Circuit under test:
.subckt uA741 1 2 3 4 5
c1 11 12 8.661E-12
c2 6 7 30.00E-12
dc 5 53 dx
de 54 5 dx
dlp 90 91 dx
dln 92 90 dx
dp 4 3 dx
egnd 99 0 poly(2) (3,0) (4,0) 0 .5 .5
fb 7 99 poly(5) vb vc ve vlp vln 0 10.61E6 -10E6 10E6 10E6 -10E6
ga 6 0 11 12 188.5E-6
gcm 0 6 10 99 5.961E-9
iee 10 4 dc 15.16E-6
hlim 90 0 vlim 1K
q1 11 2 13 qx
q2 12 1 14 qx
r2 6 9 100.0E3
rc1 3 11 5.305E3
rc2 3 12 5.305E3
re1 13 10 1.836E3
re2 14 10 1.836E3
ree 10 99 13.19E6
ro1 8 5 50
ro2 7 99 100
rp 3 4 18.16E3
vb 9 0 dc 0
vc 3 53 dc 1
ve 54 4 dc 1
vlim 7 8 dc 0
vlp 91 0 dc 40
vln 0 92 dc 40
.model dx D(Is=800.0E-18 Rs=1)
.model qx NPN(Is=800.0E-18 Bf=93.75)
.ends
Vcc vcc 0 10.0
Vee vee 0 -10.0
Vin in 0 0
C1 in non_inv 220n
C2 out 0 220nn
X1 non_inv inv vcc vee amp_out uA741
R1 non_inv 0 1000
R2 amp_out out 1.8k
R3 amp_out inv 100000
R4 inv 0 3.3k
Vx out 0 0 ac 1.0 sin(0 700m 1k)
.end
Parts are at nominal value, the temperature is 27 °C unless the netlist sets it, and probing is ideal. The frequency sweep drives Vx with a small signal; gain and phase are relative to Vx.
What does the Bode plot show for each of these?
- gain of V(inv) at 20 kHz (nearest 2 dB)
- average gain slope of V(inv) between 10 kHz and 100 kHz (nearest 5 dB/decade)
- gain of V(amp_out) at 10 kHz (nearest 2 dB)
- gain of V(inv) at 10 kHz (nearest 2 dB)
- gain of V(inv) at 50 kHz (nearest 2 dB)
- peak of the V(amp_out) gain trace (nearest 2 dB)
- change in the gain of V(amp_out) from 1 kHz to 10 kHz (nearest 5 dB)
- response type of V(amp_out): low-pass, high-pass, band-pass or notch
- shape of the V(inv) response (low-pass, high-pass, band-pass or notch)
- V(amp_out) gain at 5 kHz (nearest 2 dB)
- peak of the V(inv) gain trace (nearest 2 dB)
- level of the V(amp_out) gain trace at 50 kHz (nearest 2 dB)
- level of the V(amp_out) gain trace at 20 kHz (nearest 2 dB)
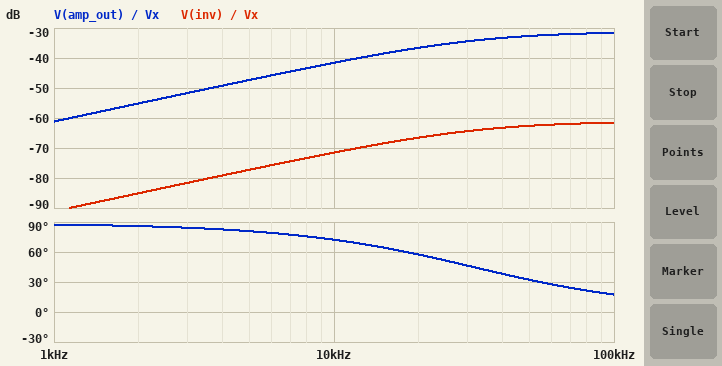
-66 dB
10 dB/decade
-42 dB
-72 dB
-62 dB
-32 dB
20 dB
high-pass
high-pass
-48 dB
-62 dB
-32 dB
-36 dB
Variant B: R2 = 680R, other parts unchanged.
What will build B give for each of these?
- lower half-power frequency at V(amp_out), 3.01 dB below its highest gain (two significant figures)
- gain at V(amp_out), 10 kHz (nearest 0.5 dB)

30 kHz
-33.0 dB
